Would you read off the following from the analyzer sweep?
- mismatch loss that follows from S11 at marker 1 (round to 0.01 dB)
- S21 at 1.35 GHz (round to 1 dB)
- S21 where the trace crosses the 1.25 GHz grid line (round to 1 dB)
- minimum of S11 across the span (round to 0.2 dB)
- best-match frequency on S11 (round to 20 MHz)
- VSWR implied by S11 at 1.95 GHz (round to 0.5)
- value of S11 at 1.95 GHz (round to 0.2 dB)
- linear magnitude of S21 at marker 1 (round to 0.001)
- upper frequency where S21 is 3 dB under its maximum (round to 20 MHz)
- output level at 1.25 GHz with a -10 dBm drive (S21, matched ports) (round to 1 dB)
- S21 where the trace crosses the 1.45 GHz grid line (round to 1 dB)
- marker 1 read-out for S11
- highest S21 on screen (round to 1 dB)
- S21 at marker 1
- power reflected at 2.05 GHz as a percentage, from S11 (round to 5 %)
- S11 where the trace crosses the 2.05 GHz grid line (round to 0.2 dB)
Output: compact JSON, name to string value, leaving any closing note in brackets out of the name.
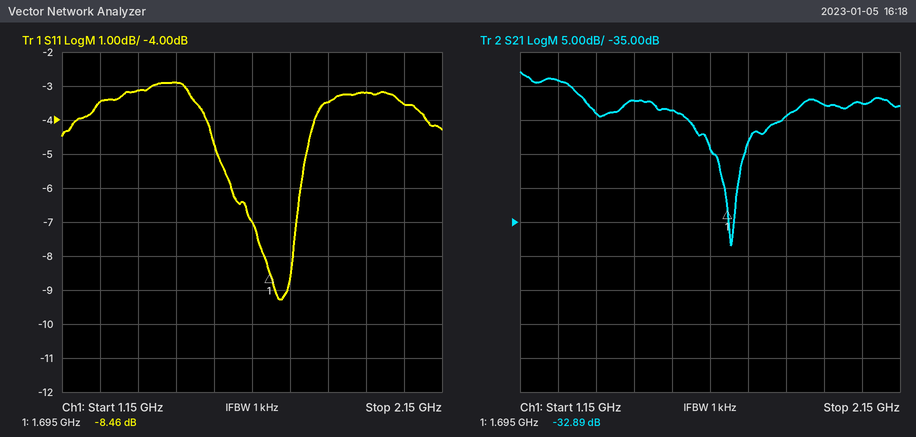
{"mismatch loss that follows from S11 at marker 1": "0.67 dB", "S21 at 1.35 GHz": "-19 dB", "S21 where the trace crosses the 1.25 GHz grid line": "-14 dB", "minimum of S11 across the span": "-9.2 dB", "best-match frequency on S11": "1.72 GHz", "VSWR implied by S11 at 1.95 GHz": "5.5", "value of S11 at 1.95 GHz": "-3.2 dB", "linear magnitude of S21 at marker 1": "0.023", "upper frequency where S21 is 3 dB under its maximum": "1.30 GHz", "output level at 1.25 GHz with a -10 dBm drive (S21, matched ports)": "-24 dBm", "S21 where the trace crosses the 1.45 GHz grid line": "-17 dB", "marker 1 read-out for S11": "-8.46 dB", "highest S21 on screen": "-13 dB", "S21 at marker 1": "-32.89 dB", "power reflected at 2.05 GHz as a percentage, from S11": "45 %", "S11 where the trace crosses the 2.05 GHz grid line": "-3.6 dB"}
